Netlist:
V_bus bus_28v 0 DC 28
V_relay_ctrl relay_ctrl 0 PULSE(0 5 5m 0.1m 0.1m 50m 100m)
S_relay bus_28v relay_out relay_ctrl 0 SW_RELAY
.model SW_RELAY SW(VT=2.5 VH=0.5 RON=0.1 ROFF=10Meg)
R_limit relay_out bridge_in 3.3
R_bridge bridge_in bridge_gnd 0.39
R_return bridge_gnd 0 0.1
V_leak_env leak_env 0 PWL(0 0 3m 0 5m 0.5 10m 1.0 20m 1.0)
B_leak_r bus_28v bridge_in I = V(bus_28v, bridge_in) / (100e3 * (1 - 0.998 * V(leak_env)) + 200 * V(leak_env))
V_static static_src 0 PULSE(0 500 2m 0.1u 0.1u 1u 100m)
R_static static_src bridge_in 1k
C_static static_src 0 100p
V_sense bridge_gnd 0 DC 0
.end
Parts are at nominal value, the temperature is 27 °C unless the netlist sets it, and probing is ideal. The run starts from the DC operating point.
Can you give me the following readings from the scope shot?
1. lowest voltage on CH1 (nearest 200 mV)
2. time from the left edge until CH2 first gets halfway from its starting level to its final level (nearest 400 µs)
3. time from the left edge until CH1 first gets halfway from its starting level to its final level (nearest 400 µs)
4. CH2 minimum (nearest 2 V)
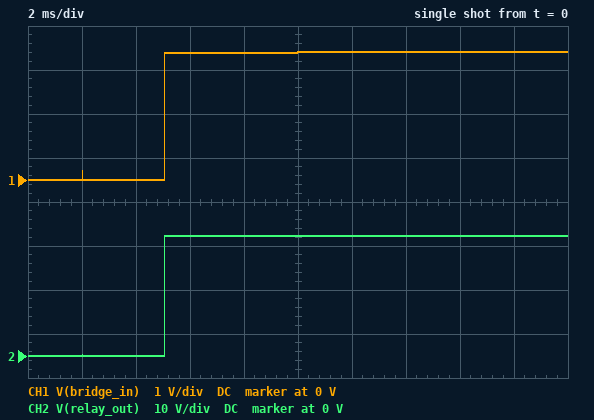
0 V
5.2 ms
5.2 ms
0 V
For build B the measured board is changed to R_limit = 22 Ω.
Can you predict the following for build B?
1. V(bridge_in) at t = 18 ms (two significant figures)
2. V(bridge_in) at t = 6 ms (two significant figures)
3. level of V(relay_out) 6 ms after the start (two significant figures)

510 mV
490 mV
28 V
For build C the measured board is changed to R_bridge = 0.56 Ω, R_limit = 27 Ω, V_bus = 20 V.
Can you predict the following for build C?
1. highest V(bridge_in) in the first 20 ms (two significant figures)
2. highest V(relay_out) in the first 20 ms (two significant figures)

430 mV
20 V
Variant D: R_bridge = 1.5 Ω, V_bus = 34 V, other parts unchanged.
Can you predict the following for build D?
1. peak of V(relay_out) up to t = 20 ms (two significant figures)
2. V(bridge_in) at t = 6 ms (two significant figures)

33 V
10 V
